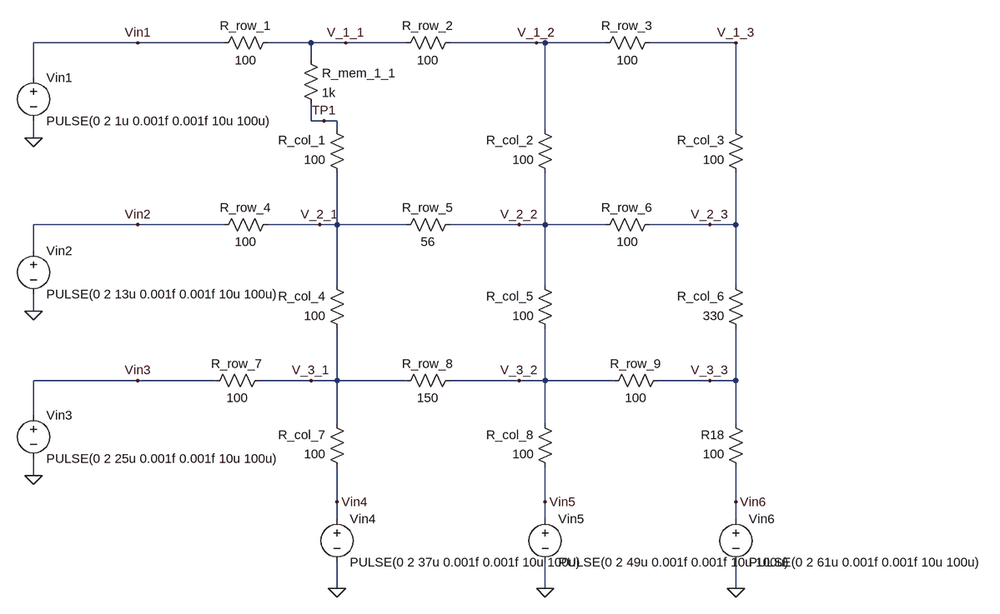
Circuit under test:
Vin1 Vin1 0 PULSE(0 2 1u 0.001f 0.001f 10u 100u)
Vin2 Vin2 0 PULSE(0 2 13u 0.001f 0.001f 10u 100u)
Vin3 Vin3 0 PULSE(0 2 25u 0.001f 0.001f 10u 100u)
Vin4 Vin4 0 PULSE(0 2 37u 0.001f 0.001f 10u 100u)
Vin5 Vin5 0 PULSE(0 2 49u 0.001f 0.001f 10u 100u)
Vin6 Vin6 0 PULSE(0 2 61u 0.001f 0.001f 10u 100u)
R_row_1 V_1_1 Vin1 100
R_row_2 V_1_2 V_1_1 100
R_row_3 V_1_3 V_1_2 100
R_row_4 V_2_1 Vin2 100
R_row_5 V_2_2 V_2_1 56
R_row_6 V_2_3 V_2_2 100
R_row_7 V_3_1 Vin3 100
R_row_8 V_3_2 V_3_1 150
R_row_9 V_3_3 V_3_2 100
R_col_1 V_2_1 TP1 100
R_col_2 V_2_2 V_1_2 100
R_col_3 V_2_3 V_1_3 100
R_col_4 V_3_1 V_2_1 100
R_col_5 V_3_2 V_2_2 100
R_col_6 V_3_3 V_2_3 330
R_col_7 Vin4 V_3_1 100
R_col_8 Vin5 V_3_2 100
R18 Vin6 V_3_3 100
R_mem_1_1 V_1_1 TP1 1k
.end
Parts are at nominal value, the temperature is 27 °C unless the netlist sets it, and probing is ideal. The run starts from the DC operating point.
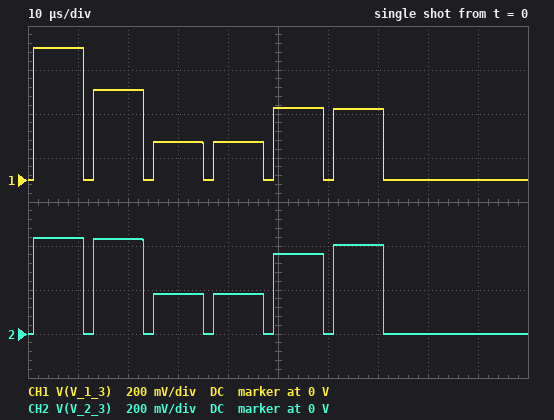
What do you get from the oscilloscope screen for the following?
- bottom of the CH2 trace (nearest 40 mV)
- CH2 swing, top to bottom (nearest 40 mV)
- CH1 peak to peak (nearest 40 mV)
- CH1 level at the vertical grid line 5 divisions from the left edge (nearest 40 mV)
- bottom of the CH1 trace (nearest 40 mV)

0 V
440 mV
600 mV
320 mV
0 V
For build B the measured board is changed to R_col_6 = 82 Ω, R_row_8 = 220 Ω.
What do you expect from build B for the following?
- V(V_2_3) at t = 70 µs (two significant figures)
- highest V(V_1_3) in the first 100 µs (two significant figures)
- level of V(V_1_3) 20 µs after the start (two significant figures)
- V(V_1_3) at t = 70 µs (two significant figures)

640 mV
530 mV
340 mV
490 mV
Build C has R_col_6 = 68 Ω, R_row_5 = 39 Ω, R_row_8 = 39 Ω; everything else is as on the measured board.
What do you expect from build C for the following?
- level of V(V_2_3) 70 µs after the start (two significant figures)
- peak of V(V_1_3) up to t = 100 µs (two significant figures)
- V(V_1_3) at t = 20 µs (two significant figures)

630 mV
500 mV
360 mV
